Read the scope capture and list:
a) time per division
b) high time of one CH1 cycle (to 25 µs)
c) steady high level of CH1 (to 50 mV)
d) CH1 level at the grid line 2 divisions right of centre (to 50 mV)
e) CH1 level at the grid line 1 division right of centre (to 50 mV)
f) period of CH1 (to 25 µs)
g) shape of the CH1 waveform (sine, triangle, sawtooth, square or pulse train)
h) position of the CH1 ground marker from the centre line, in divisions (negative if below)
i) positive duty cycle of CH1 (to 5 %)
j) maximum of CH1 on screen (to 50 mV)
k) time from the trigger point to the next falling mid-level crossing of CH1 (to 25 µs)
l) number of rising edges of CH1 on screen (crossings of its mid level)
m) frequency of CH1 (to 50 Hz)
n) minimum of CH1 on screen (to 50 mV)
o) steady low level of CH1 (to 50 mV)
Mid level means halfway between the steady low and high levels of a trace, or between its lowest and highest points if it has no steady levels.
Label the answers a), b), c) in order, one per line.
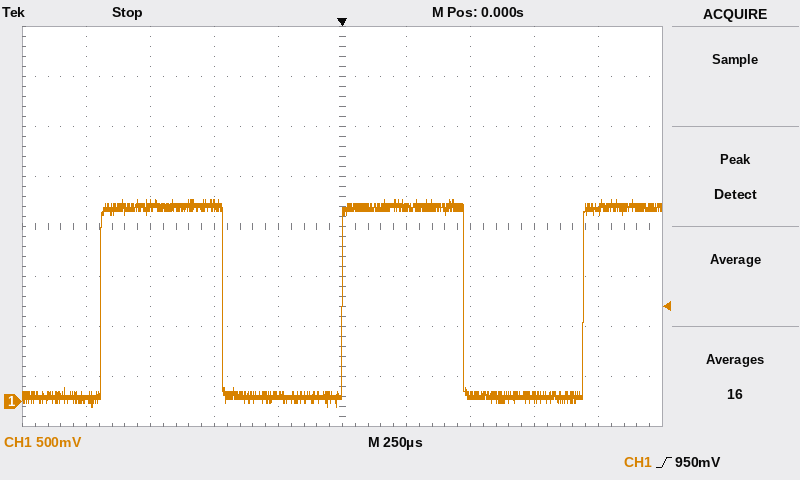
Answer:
a) 250 µs
b) 475 µs
c) 1.95 V
d) 50 mV
e) 1.95 V
f) 950 µs
g) square
h) -3.5 div
i) 50 %
j) 2.00 V
k) 475 µs
l) 3
m) 1.05 kHz
n) -50 mV
o) 50 mV
